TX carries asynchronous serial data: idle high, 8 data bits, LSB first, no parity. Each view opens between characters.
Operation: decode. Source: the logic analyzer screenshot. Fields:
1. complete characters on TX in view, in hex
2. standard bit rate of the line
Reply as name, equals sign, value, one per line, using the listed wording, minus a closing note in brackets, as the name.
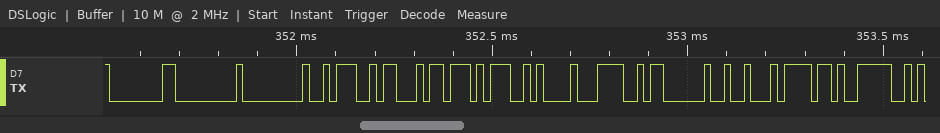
complete characters on TX in view, in hex = 80, 00, 00, 3A, A3, D7, 0A, 3C, 03, 12, 6F, 3E
standard bit rate of the line = 57600 baud
